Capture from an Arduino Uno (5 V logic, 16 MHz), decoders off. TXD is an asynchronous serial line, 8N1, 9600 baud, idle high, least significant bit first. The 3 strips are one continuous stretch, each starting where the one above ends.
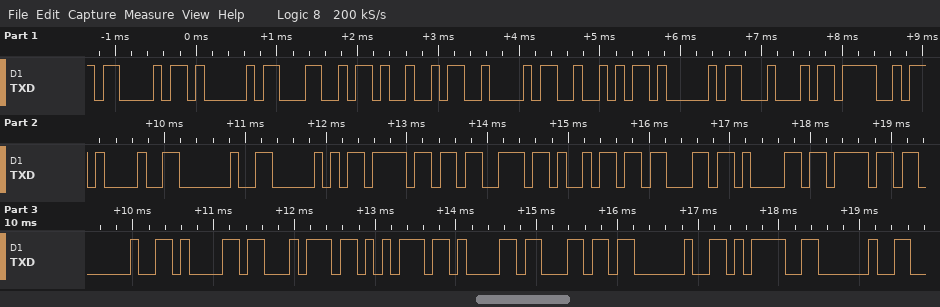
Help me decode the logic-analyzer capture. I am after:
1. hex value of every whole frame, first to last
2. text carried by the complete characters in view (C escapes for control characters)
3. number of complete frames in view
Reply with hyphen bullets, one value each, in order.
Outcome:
- 43 41 4C 49 42 52 41 44 4F 21 20 50 6F 73 69 63 61 6F 20 61 74 75 61 6C 20 3D 20
- "CALIBRADO! Posicao atual = "
- 27
